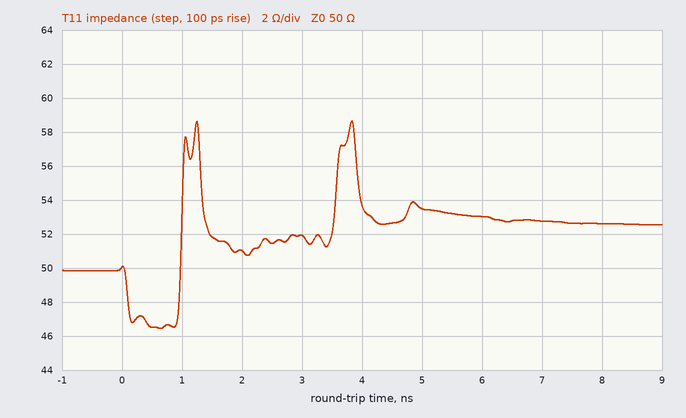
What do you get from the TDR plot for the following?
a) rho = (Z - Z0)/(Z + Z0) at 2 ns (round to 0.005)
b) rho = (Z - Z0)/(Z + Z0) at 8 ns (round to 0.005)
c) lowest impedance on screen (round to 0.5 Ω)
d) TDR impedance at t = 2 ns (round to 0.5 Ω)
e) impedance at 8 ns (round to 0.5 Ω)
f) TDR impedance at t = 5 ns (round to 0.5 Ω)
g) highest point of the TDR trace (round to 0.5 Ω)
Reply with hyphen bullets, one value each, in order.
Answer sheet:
- +0.010
- +0.025
- 46.5 Ω
- 51.0 Ω
- 52.5 Ω
- 53.5 Ω
- 58.5 Ω
